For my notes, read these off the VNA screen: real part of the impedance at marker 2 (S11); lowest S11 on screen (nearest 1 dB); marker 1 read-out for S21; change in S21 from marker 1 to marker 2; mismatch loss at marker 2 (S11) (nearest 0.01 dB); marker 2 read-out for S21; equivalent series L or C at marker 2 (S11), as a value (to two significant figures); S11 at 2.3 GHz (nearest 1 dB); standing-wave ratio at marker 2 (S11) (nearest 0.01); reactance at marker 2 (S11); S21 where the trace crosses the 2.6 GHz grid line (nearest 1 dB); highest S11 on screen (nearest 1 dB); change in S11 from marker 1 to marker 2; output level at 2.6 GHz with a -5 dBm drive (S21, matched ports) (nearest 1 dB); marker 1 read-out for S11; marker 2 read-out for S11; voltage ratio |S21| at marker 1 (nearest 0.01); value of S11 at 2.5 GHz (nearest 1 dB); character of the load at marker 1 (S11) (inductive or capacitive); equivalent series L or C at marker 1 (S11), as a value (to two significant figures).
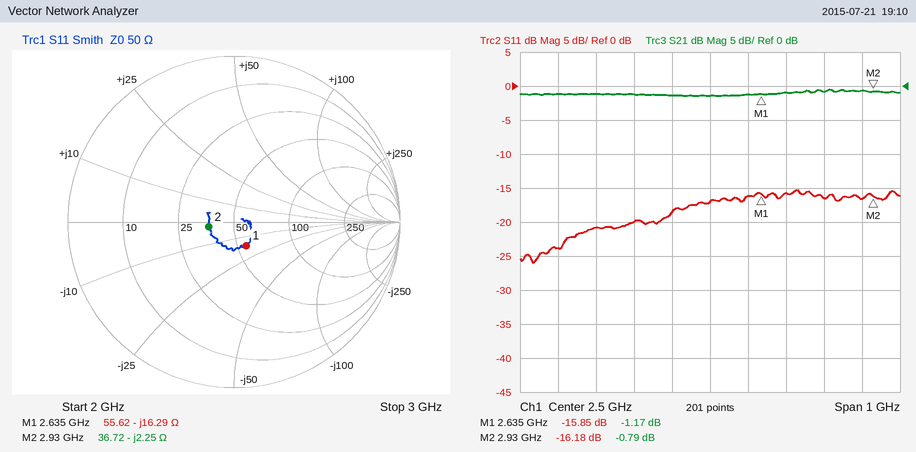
36.72 Ω
-26 dB
-1.17 dB
0.38 dB
0.11 dB
-0.79 dB
24 pF
-20 dB
1.37
-2.25 Ω
-1 dB
-15 dB
-0.33 dB
-6 dBm
-15.85 dB
-16.18 dB
0.87
-17 dB
capacitive
3.7 pF
